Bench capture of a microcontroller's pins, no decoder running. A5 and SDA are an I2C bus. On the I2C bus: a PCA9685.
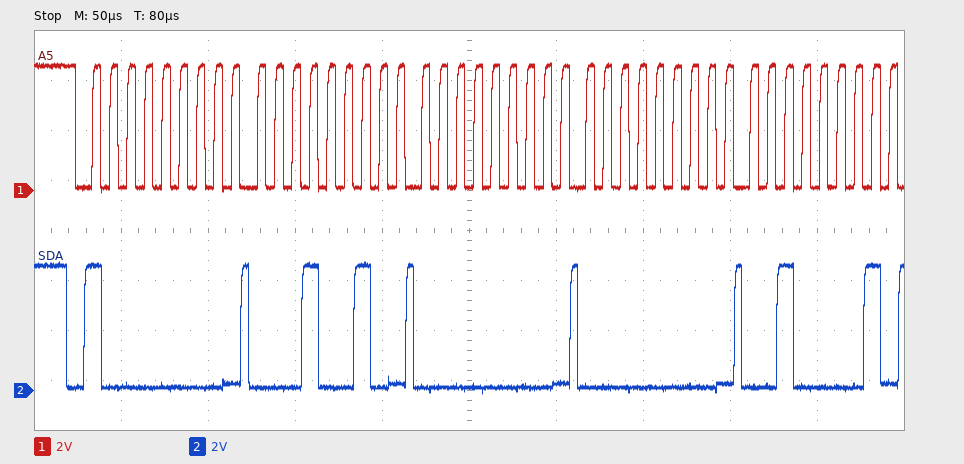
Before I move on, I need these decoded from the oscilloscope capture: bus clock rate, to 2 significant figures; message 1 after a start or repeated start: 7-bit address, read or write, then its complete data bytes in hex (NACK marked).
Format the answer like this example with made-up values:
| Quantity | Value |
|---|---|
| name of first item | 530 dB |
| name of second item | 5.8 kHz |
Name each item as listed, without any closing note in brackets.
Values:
| Quantity | Value |
|---|---|
| bus clock rate, to 2 significant figures | 100 kHz |
| message 1 after a start or repeated start: 7-bit address, read or write, then its complete data bytes in hex | 0x40 write: 12 00 00 21 |
